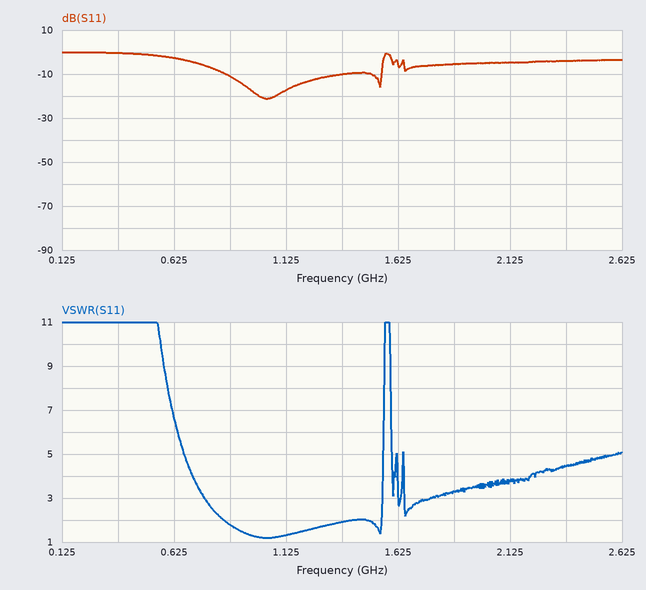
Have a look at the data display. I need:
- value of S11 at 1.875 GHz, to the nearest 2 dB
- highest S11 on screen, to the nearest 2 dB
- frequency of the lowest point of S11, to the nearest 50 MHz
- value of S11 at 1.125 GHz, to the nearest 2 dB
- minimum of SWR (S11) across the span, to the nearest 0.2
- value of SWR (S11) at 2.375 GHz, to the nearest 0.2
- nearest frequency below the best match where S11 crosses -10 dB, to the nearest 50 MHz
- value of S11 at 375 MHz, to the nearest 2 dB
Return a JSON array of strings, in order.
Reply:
["-6 dB", "0 dB", "1.05 GHz", "-18 dB", "1.2", "4.4", "850 MHz", "0 dB"]
